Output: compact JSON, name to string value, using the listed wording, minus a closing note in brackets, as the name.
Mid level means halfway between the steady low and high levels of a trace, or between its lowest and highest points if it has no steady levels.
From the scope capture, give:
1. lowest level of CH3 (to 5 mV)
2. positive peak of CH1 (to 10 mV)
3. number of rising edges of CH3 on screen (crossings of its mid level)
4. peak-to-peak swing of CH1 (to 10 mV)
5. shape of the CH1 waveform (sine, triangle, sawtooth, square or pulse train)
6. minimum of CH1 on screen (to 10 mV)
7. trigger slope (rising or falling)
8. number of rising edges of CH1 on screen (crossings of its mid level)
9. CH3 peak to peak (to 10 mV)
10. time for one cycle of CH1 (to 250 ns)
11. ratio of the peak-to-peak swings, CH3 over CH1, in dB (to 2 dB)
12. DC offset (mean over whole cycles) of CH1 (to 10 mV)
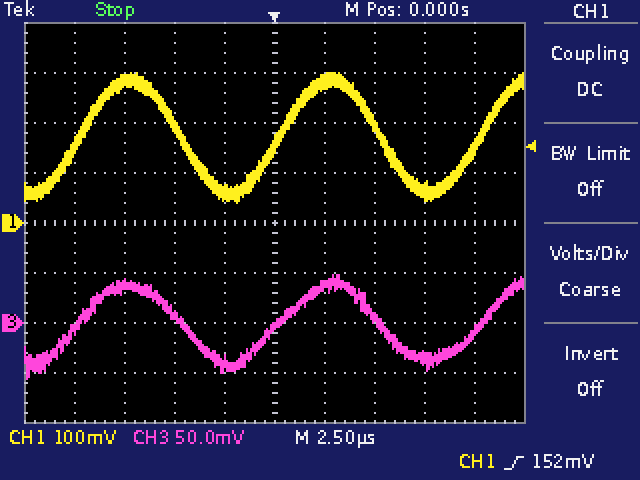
{"lowest level of CH3": "-55 mV", "positive peak of CH1": "300 mV", "number of rising edges of CH3 on screen": "3", "peak-to-peak swing of CH1": "260 mV", "shape of the CH1 waveform": "sine", "minimum of CH1 on screen": "40 mV", "trigger slope": "rising", "number of rising edges of CH1 on screen": "3", "CH3 peak to peak": "100 mV", "time for one cycle of CH1": "10.00 µs", "ratio of the peak-to-peak swings, CH3 over CH1, in dB": "-8 dB", "DC offset (mean over whole cycles) of CH1": "170 mV"}
